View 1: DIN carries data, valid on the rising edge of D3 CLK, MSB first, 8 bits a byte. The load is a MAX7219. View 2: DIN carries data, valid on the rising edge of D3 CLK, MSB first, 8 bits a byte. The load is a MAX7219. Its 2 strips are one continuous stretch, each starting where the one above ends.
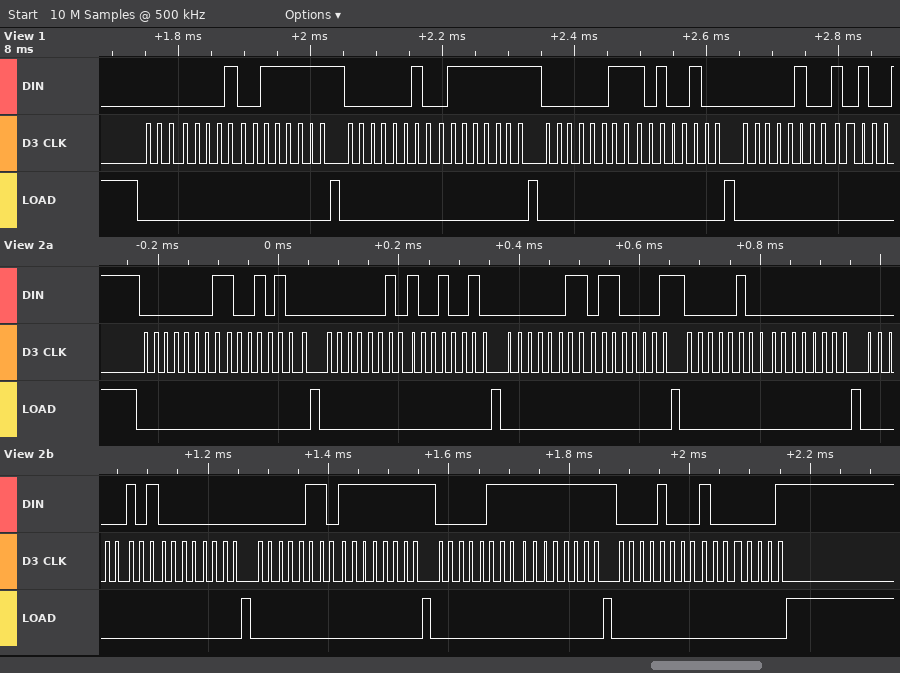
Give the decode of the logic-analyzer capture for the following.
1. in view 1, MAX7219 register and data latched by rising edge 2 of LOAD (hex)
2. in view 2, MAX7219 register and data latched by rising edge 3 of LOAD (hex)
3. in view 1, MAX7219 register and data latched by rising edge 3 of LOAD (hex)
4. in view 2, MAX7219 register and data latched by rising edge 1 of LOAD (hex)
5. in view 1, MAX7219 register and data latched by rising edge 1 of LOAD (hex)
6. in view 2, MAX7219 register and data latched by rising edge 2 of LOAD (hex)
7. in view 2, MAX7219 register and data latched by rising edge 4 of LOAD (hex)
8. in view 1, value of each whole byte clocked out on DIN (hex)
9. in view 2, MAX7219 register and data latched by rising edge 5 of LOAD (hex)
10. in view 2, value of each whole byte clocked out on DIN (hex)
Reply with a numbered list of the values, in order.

1. register 0x2, data 0x7F
2. register 0x3, data 0x61
3. register 0x3, data 0xA4
4. register 0x1, data 0x94
5. register 0x1, data 0x3F
6. register 0x2, data 0x92
7. register 0x4, data 0x00
8. 0x01 0x3F 0x02 0x7F 0x03 0xA4 0x04
9. register 0x5, data 0x00
10. 01 94 02 92 03 61 04 00 05 00 06 FF 07 FF 08 81
